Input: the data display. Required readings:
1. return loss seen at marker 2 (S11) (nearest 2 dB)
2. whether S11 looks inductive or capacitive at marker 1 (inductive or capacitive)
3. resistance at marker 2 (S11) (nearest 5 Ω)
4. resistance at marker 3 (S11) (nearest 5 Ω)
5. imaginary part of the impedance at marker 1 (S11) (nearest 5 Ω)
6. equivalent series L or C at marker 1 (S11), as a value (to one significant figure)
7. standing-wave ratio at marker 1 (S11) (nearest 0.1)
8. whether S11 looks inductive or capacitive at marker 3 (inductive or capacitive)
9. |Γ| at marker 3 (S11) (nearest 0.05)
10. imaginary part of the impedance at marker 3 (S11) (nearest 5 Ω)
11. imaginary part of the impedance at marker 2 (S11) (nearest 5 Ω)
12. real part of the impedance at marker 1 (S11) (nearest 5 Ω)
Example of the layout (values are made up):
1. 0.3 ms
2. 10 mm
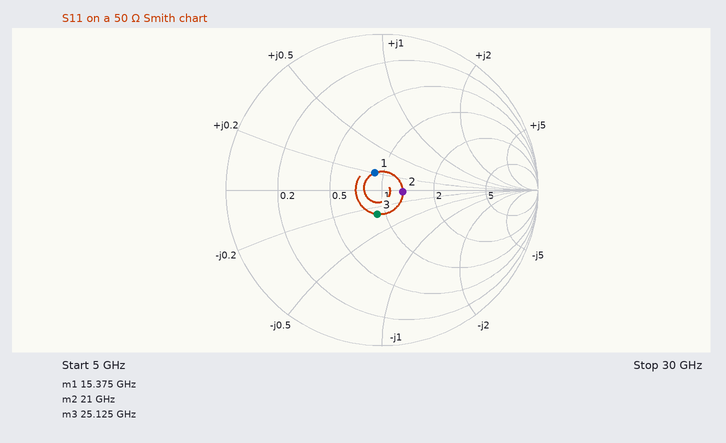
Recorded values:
1. 18 dB
2. inductive
3. 65 Ω
4. 45 Ω
5. +10 Ω
6. 100 pH
7. 1.3
8. capacitive
9. 0.15
10. -15 Ω
11. 0 Ω
12. 45 Ω
